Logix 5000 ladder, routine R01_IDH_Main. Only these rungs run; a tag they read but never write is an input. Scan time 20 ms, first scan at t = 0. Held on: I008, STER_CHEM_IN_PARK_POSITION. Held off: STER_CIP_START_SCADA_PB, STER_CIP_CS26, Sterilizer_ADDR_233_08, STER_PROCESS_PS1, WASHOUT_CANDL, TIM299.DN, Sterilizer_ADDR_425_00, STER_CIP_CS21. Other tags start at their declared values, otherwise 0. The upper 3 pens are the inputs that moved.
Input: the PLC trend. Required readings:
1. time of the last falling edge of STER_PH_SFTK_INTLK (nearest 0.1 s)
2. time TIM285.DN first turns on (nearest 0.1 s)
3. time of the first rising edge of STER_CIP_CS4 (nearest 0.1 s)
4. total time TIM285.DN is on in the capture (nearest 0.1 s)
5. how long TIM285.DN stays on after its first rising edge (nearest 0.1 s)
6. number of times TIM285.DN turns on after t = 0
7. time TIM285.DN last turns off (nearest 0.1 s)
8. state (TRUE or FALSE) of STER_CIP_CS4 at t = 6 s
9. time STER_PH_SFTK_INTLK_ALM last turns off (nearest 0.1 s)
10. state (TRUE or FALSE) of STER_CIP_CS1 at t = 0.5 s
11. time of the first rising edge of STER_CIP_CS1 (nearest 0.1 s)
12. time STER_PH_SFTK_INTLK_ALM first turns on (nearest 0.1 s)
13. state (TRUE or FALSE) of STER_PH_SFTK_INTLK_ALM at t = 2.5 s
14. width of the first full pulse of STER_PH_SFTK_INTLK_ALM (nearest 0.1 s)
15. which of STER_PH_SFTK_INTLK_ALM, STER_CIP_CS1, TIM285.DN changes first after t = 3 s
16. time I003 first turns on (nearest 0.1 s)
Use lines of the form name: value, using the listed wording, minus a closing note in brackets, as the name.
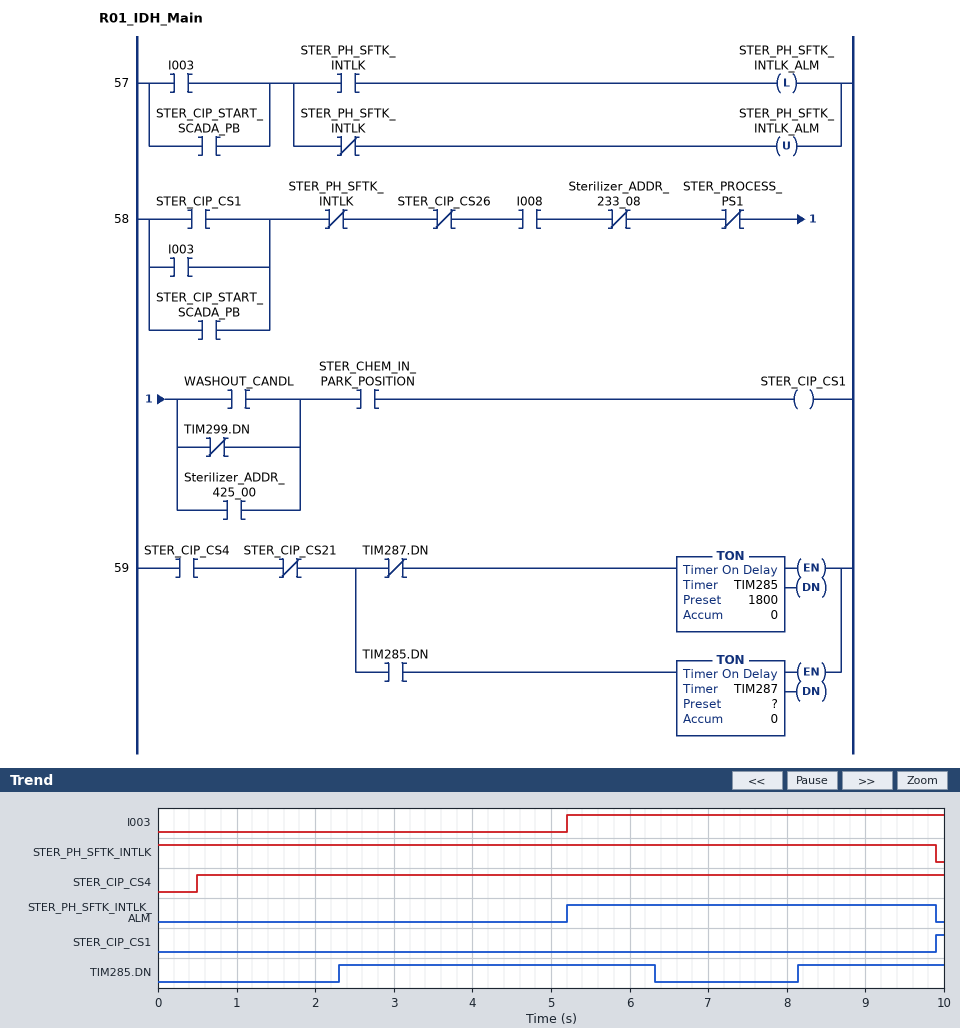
time of the last falling edge of STER_PH_SFTK_INTLK: 9.9 s
time TIM285.DN first turns on: 2.3 s
time of the first rising edge of STER_CIP_CS4: 0.5 s
total time TIM285.DN is on in the capture: 5.9 s
how long TIM285.DN stays on after its first rising edge: 4.0 s
number of times TIM285.DN turns on after t = 0: 2
time TIM285.DN last turns off: 6.3 s
state (TRUE or FALSE) of STER_CIP_CS4 at t = 6 s: TRUE
time STER_PH_SFTK_INTLK_ALM last turns off: 9.9 s
state (TRUE or FALSE) of STER_CIP_CS1 at t = 0.5 s: FALSE
time of the first rising edge of STER_CIP_CS1: 9.9 s
time STER_PH_SFTK_INTLK_ALM first turns on: 5.2 s
state (TRUE or FALSE) of STER_PH_SFTK_INTLK_ALM at t = 2.5 s: FALSE
width of the first full pulse of STER_PH_SFTK_INTLK_ALM: 4.7 s
which of STER_PH_SFTK_INTLK_ALM, STER_CIP_CS1, TIM285.DN changes first after t = 3 s: STER_PH_SFTK_INTLK_ALM
time I003 first turns on: 5.2 s
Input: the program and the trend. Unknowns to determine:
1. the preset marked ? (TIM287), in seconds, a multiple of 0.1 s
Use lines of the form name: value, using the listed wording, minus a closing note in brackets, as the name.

the preset marked ? (TIM287), in seconds, a multiple of 0.1 s: 4.0 s
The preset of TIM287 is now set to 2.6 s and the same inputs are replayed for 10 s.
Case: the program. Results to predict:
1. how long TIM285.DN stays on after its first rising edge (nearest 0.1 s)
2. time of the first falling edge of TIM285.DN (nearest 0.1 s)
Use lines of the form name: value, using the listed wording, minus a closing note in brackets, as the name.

how long TIM285.DN stays on after its first rising edge: 2.6 s
time of the first falling edge of TIM285.DN: 4.9 s
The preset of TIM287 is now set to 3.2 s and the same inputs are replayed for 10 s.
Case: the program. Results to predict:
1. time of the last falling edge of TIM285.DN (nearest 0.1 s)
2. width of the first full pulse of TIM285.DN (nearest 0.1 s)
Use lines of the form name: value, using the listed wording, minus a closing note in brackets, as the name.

time of the last falling edge of TIM285.DN: 5.5 s
width of the first full pulse of TIM285.DN: 3.2 s
